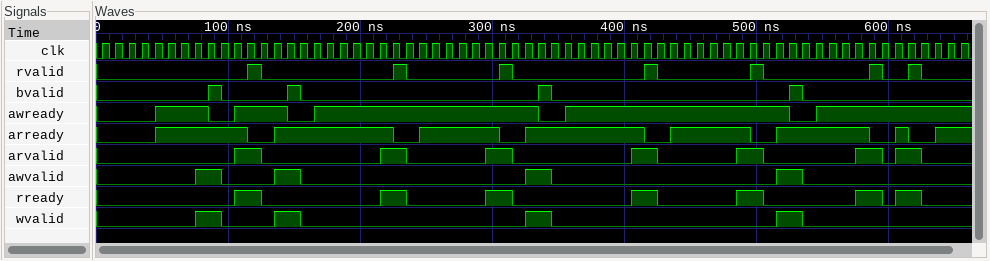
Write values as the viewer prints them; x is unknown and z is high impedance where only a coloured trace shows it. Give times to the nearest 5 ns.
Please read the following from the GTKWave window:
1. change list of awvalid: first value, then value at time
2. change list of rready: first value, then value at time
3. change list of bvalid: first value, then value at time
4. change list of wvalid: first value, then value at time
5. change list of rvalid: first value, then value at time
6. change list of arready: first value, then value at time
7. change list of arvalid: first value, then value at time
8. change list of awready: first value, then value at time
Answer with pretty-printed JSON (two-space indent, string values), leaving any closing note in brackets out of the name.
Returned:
{
  "change list of awvalid: first value, then value at time": "0, 1 at 75 ns, 0 at 95 ns, 1 at 135 ns, 0 at 155 ns, 1 at 325 ns, 0 at 345 ns, 1 at 515 ns, 0 at 535 ns",
  "change list of rready: first value, then value at time": "0, 1 at 105 ns, 0 at 125 ns, 1 at 215 ns, 0 at 235 ns, 1 at 295 ns, 0 at 315 ns, 1 at 405 ns, 0 at 425 ns, 1 at 485 ns, 0 at 505 ns, 1 at 575 ns, 0 at 595 ns, 1 at 605 ns, 0 at 625 ns",
  "change list of bvalid: first value, then value at time": "0, 1 at 85 ns, 0 at 95 ns, 1 at 145 ns, 0 at 155 ns, 1 at 335 ns, 0 at 345 ns, 1 at 525 ns, 0 at 535 ns",
  "change list of wvalid: first value, then value at time": "0, 1 at 75 ns, 0 at 95 ns, 1 at 135 ns, 0 at 155 ns, 1 at 325 ns, 0 at 345 ns, 1 at 515 ns, 0 at 535 ns",
  "change list of rvalid: first value, then value at time": "0, 1 at 115 ns, 0 at 125 ns, 1 at 225 ns, 0 at 235 ns, 1 at 305 ns, 0 at 315 ns, 1 at 415 ns, 0 at 425 ns, 1 at 495 ns, 0 at 505 ns, 1 at 585 ns, 0 at 595 ns, 1 at 615 ns, 0 at 625 ns",
  "change list of arready: first value, then value at time": "0, 1 at 45 ns, 0 at 115 ns, 1 at 135 ns, 0 at 225 ns, 1 at 245 ns, 0 at 305 ns, 1 at 325 ns, 0 at 415 ns, 1 at 435 ns, 0 at 495 ns, 1 at 515 ns, 0 at 585 ns, 1 at 605 ns, 0 at 615 ns, 1 at 635 ns",
  "change list of arvalid: first value, then value at time": "0, 1 at 105 ns, 0 at 125 ns, 1 at 215 ns, 0 at 235 ns, 1 at 295 ns, 0 at 315 ns, 1 at 405 ns, 0 at 425 ns, 1 at 485 ns, 0 at 505 ns, 1 at 575 ns, 0 at 595 ns, 1 at 605 ns, 0 at 625 ns",
  "change list of awready: first value, then value at time": "0, 1 at 45 ns, 0 at 85 ns, 1 at 105 ns, 0 at 145 ns, 1 at 165 ns, 0 at 335 ns, 1 at 355 ns, 0 at 525 ns, 1 at 545 ns"
}
